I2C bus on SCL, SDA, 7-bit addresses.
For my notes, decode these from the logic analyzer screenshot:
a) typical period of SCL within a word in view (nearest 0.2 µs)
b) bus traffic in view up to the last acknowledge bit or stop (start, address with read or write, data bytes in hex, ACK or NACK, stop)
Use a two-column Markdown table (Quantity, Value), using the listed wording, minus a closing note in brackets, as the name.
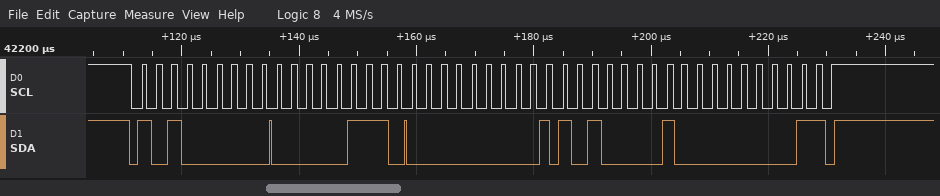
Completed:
| Quantity | Value |
|---|---|
| typical period of SCL within a word in view | 2.6 µs |
| bus traffic in view up to the last acknowledge bit or stop | start, address 50 write ACK, 07 ACK, 00 ACK, repeated start, address 50 read ACK, 01 NACK, stop |
